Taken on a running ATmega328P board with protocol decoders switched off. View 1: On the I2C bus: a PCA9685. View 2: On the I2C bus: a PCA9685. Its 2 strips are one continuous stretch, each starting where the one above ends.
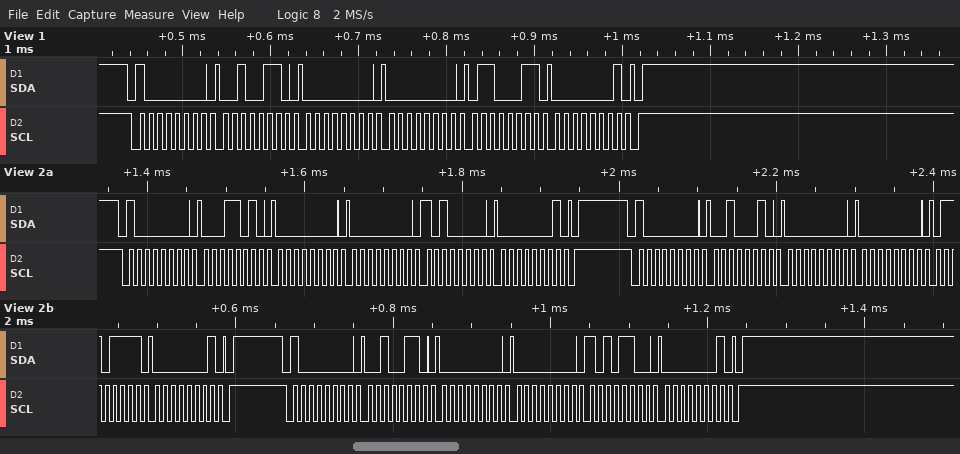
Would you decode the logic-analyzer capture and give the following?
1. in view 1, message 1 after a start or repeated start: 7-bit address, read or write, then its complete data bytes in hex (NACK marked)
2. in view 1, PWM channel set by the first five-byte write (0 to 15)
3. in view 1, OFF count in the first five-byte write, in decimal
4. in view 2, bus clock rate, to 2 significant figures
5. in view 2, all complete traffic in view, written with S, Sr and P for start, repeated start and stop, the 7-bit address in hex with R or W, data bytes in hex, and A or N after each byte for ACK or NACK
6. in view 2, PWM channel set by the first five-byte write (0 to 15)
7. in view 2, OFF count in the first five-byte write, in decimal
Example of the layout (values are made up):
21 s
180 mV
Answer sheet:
0x40 write: 26 00 00 63 01
8
355
100 kHz
S 40W A 1A A 00 A 00 A A0 A 01 A P S 40W A 22 A 00 A 00 A 6F A 01 A P S 40W A 26 A 00 A 00 A AC A 01 A P
5
416
